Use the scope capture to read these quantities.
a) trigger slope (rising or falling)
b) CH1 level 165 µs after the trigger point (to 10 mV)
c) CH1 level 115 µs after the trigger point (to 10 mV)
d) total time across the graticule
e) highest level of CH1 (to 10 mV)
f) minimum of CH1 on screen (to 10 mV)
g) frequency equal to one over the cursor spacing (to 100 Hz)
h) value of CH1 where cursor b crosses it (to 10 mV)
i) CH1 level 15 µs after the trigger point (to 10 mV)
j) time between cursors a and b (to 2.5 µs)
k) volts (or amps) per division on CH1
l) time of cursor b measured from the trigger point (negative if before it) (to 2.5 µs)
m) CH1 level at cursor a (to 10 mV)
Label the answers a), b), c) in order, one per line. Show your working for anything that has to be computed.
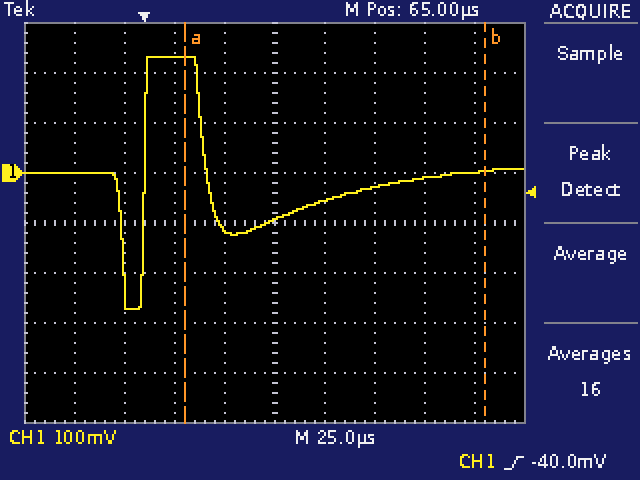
a) rising
b) 0 mV
c) -30 mV
d) 250 µs
e) 230 mV
f) -270 mV
g) 1 / 150.0 µs ≈ 6.7 kHz
h) 0 mV
i) 230 mV
j) 150.0 µs
k) 100 mV
l) +170.0 µs
m) 230 mV
